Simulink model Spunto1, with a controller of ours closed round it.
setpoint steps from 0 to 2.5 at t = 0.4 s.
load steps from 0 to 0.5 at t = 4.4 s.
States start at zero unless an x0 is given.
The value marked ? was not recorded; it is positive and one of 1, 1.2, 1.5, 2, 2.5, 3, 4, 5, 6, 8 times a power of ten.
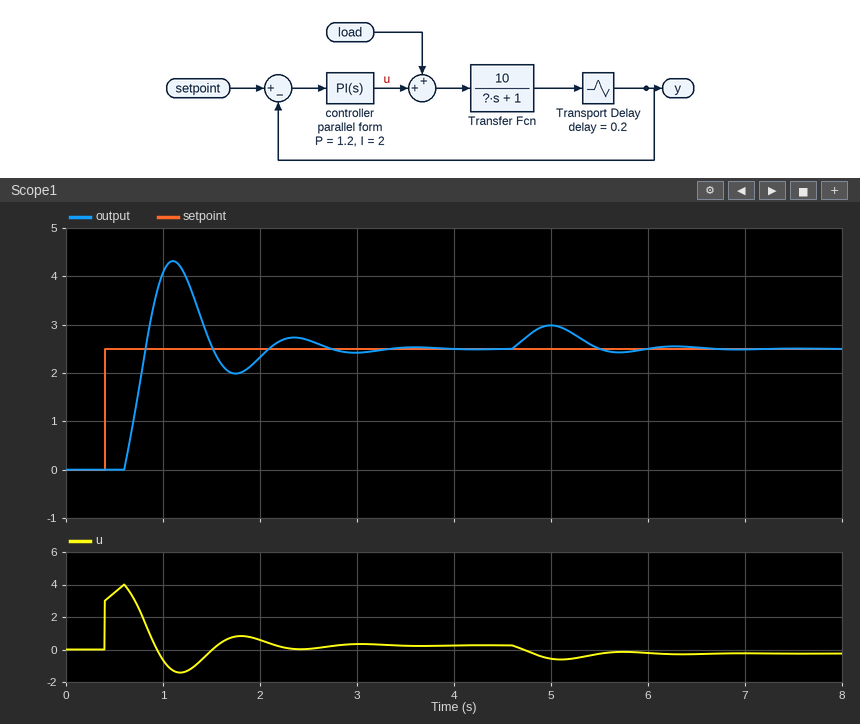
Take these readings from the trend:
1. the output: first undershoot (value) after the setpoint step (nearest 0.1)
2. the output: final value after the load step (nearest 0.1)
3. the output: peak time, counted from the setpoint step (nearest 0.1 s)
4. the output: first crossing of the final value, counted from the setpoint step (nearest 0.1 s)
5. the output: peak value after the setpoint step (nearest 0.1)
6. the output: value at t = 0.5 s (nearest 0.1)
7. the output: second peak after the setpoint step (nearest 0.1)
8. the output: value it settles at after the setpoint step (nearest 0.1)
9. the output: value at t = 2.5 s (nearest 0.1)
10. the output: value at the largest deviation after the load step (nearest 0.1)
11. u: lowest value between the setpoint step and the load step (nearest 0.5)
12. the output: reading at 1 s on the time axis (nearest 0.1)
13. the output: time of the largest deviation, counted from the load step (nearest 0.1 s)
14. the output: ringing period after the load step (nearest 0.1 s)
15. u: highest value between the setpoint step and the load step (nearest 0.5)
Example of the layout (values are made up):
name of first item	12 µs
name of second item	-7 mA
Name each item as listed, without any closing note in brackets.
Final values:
the output: first undershoot (value) after the setpoint step	2.0
the output: final value after the load step	2.5
the output: peak time, counted from the setpoint step	0.7 s
the output: first crossing of the final value, counted from the setpoint step	0.4 s
the output: peak value after the setpoint step	4.3
the output: value at t = 0.5 s	0.0
the output: second peak after the setpoint step	2.7
the output: value it settles at after the setpoint step	2.5
the output: value at t = 2.5 s	2.7
the output: value at the largest deviation after the load step	3.0
u: lowest value between the setpoint step and the load step	-1.5
the output: reading at 1 s on the time axis	4.1
the output: time of the largest deviation, counted from the load step	0.6 s
the output: ringing period after the load step	1.3 s
u: highest value between the setpoint step and the load step	4.0
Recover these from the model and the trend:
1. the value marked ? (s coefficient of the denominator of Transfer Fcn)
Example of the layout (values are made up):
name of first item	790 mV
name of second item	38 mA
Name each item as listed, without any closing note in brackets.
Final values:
the value marked ?	3
